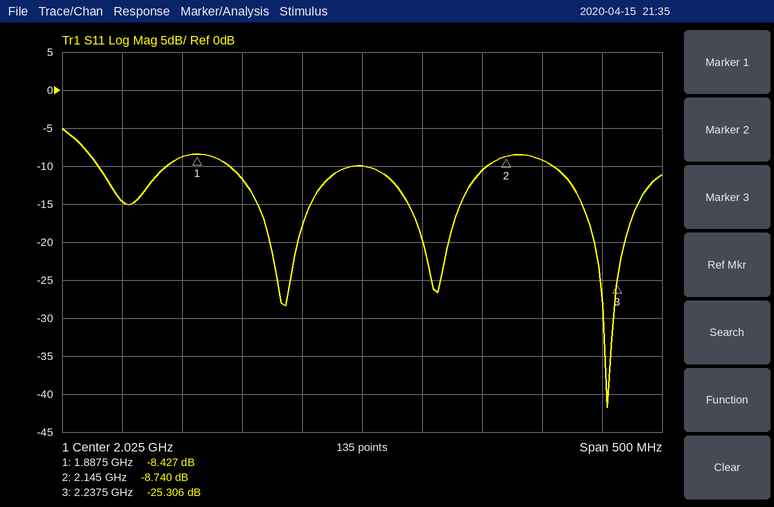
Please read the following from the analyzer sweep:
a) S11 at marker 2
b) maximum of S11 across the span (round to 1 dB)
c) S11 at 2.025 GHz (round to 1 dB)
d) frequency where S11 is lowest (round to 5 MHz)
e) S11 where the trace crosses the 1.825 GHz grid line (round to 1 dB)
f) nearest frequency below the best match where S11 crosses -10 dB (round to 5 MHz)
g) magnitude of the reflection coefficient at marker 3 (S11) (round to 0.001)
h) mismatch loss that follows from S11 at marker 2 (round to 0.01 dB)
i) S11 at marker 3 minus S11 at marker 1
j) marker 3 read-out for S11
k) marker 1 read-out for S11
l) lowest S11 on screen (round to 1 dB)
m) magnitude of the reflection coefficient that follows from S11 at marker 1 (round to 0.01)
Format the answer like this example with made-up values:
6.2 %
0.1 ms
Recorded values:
-8.740 dB
-5 dB
-10 dB
2.230 GHz
-15 dB
2.185 GHz
0.054
0.62 dB
-16.879 dB
-25.306 dB
-8.427 dB
-42 dB
0.38
